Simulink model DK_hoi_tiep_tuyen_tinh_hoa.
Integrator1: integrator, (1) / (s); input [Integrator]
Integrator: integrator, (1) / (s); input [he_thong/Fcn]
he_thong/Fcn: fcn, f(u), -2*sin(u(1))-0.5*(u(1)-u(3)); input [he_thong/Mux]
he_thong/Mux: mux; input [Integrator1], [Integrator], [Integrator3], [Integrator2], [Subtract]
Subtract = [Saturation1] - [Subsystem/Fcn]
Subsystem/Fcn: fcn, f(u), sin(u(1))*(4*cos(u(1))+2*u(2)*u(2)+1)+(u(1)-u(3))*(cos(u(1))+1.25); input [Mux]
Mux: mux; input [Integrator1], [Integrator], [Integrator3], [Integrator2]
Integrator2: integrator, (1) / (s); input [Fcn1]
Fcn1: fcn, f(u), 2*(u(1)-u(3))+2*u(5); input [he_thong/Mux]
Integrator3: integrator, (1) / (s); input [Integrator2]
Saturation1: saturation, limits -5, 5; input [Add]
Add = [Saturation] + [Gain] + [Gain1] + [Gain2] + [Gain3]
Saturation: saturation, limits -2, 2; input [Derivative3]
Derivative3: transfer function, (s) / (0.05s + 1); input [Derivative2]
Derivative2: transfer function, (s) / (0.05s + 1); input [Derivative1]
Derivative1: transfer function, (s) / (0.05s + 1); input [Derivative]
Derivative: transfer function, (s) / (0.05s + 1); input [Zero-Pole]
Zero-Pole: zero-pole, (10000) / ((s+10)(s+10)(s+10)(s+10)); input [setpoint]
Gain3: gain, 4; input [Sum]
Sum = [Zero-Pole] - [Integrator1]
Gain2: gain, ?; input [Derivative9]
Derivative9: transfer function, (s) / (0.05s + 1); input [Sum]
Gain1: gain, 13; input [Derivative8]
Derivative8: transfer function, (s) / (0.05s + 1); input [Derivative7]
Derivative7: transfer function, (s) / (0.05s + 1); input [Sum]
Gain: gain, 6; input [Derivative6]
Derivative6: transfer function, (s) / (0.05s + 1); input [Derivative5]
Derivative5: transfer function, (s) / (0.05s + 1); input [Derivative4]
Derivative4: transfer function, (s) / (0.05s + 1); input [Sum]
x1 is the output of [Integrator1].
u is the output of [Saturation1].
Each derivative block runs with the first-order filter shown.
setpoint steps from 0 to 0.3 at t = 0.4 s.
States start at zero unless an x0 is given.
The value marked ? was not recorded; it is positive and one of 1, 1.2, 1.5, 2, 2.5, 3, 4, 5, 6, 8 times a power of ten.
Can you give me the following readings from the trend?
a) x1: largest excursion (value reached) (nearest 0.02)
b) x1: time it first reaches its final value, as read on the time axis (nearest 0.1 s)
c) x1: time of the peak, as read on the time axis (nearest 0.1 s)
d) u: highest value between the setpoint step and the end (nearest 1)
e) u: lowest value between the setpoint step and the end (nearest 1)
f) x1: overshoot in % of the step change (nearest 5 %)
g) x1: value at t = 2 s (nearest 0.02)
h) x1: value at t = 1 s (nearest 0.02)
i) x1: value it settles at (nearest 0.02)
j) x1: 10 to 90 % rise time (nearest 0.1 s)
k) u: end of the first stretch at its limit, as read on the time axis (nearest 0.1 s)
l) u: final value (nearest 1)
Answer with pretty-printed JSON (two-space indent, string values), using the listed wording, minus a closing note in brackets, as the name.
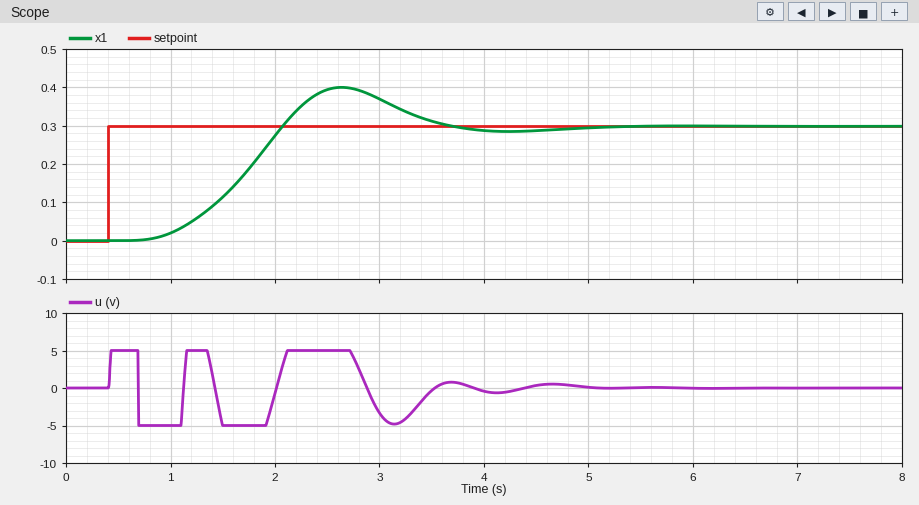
{
  "x1: largest excursion (value reached)": "0.40",
  "x1: time it first reaches its final value, as read on the time axis": "2.1 s",
  "x1: time of the peak, as read on the time axis": "2.6 s",
  "u: highest value between the setpoint step and the end": "5",
  "u: lowest value between the setpoint step and the end": "-5",
  "x1: overshoot in % of the step change": "35 %",
  "x1: value at t = 2 s": "0.28",
  "x1: value at t = 1 s": "0.02",
  "x1: value it settles at": "0.30",
  "x1: 10 to 90 % rise time": "0.9 s",
  "u: end of the first stretch at its limit, as read on the time axis": "0.7 s",
  "u: final value": "0"
}
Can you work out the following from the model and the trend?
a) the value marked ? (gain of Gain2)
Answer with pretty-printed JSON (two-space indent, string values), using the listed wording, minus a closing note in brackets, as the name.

{
  "the value marked ?": "25"
}
